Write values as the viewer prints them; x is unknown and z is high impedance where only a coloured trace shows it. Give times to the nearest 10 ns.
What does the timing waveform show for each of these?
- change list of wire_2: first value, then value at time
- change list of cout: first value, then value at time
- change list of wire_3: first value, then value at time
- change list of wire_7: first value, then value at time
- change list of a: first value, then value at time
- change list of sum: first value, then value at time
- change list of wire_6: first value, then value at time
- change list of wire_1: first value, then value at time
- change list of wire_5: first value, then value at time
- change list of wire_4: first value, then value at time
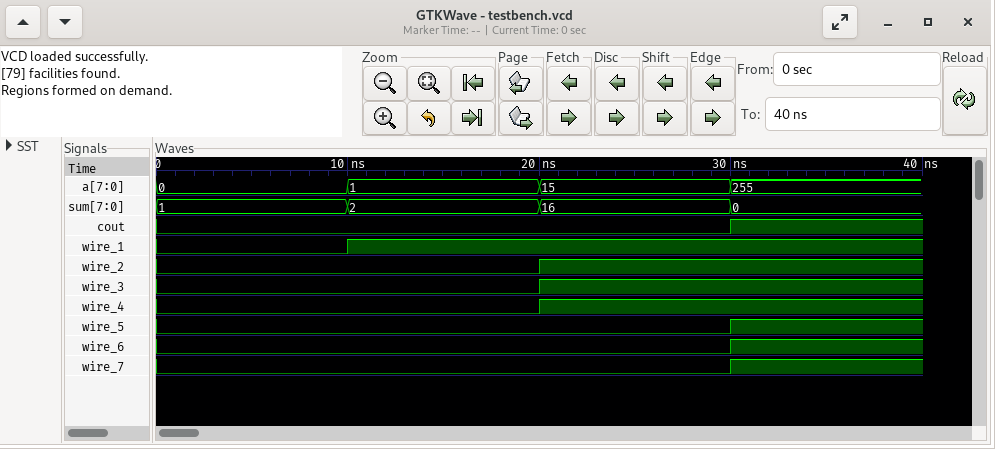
0, 1 at 20 ns
0, 1 at 30 ns
0, 1 at 20 ns
0, 1 at 30 ns
0, 1 at 10 ns, 15 at 20 ns, 255 at 30 ns
1, 2 at 10 ns, 16 at 20 ns, 0 at 30 ns
0, 1 at 30 ns
0, 1 at 10 ns
0, 1 at 30 ns
0, 1 at 20 ns
